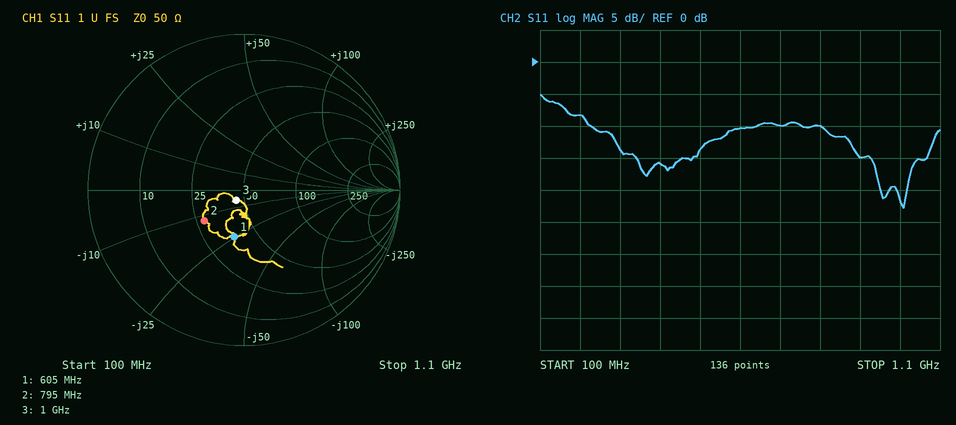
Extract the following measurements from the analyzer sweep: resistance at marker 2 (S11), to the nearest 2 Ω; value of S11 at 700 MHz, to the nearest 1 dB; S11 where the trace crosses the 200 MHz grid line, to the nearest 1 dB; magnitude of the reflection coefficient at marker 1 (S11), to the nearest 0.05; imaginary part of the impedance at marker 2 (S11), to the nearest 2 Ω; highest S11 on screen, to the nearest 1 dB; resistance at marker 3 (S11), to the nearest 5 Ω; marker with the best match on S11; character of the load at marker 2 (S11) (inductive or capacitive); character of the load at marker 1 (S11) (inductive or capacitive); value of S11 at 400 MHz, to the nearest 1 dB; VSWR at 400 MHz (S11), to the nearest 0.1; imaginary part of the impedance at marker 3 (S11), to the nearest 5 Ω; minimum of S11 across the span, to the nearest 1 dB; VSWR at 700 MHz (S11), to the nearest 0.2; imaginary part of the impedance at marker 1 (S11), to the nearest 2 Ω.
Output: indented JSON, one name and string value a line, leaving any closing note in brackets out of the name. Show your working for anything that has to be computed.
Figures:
{
  "resistance at marker 2 (S11), to the nearest 2 Ω": "28 Ω",
  "value of S11 at 700 MHz, to the nearest 1 dB": "-10 dB",
  "S11 where the trace crosses the 200 MHz grid line, to the nearest 1 dB": "-8 dB",
  "magnitude of the reflection coefficient at marker 1 (S11), to the nearest 0.05": "0.30",
  "imaginary part of the impedance at marker 2 (S11), to the nearest 2 Ω": "-12 Ω",
  "highest S11 on screen, to the nearest 1 dB": "-5 dB",
  "resistance at marker 3 (S11), to the nearest 5 Ω": "45 Ω",
  "marker with the best match on S11": "marker 3",
  "character of the load at marker 2 (S11)": "capacitive",
  "character of the load at marker 1 (S11)": "capacitive",
  "value of S11 at 400 MHz, to the nearest 1 dB": "-16 dB",
  "VSWR at 400 MHz (S11), to the nearest 0.1": "|Γ| = 10^(-16/20) = 0.1585; VSWR = (1 + 0.1585)/(1 − 0.1585) ≈ 1.4",
  "imaginary part of the impedance at marker 3 (S11), to the nearest 5 Ω": "-5 Ω",
  "minimum of S11 across the span, to the nearest 1 dB": "-23 dB",
  "VSWR at 700 MHz (S11), to the nearest 0.2": "|Γ| = 10^(-10/20) = 0.3162; VSWR = (1 + 0.3162)/(1 − 0.3162) ≈ 1.92, so 2.0 to the nearest 0.2",
  "imaginary part of the impedance at marker 1 (S11), to the nearest 2 Ω": "-24 Ω"
}
